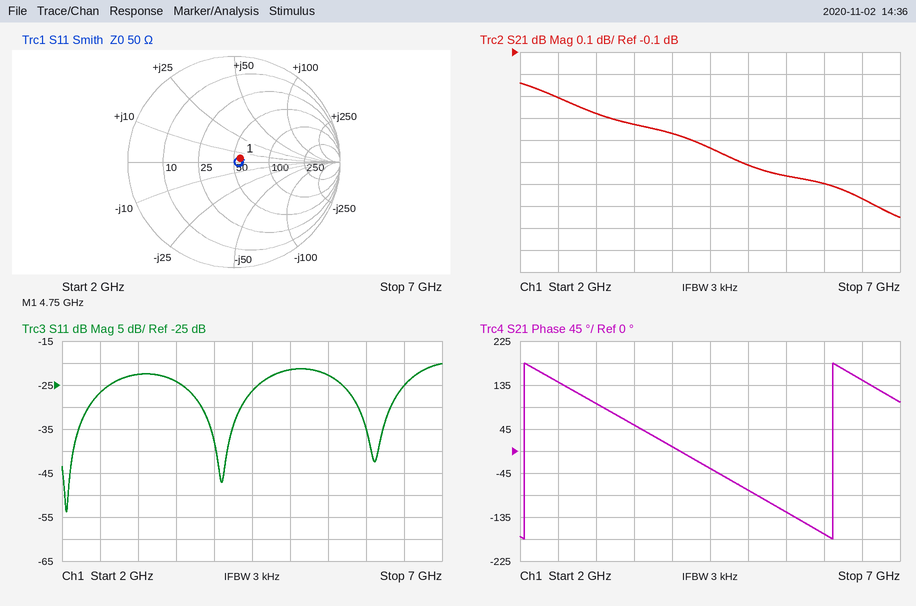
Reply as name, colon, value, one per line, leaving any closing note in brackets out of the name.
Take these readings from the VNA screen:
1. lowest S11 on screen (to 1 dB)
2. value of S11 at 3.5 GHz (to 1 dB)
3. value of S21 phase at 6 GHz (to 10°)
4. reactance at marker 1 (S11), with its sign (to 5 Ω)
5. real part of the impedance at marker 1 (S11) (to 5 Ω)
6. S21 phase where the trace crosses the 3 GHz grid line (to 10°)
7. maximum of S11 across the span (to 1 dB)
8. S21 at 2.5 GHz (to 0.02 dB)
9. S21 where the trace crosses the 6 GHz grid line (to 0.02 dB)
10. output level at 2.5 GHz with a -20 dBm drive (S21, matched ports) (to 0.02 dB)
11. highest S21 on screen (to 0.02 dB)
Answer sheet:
lowest S11 on screen: -54 dB
value of S11 at 3.5 GHz: -24 dB
value of S21 phase at 6 GHz: -170°
reactance at marker 1 (S11), with its sign: +5 Ω
real part of the impedance at marker 1 (S11): 55 Ω
S21 phase where the trace crosses the 3 GHz grid line: 100°
maximum of S11 across the span: -20 dB
S21 at 2.5 GHz: -0.30 dB
S21 where the trace crosses the 6 GHz grid line: -0.70 dB
output level at 2.5 GHz with a -20 dBm drive (S21, matched ports): -20.30 dBm
highest S21 on screen: -0.24 dB
